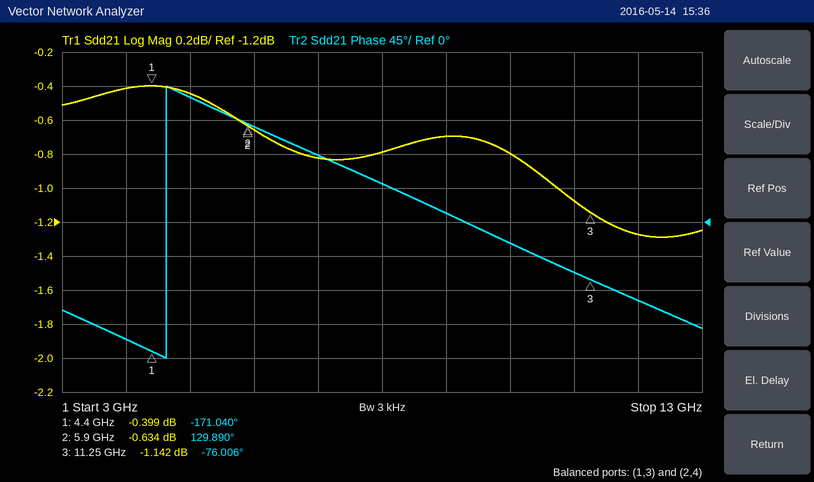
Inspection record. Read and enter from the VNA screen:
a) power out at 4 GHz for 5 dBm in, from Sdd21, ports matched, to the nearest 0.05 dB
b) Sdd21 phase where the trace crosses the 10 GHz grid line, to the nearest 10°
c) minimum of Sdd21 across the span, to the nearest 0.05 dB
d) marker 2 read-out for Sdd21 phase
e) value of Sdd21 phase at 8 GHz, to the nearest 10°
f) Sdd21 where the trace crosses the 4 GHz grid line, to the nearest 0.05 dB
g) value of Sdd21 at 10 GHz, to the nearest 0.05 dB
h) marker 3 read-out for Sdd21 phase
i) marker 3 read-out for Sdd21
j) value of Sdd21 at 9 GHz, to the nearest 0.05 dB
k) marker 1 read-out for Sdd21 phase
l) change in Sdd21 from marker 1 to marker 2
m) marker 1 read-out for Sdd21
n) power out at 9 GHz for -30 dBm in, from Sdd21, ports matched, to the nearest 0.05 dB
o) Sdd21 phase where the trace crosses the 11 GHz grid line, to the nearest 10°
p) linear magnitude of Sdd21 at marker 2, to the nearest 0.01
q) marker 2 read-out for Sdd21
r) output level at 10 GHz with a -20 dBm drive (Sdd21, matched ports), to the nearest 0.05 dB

4.60 dBm
-30°
-1.30 dB
129.890°
50°
-0.40 dB
-0.80 dB
-76.006°
-1.142 dB
-0.70 dB
-171.040°
-0.235 dB
-0.399 dB
-30.70 dBm
-70°
0.93
-0.634 dB
-20.80 dBm
